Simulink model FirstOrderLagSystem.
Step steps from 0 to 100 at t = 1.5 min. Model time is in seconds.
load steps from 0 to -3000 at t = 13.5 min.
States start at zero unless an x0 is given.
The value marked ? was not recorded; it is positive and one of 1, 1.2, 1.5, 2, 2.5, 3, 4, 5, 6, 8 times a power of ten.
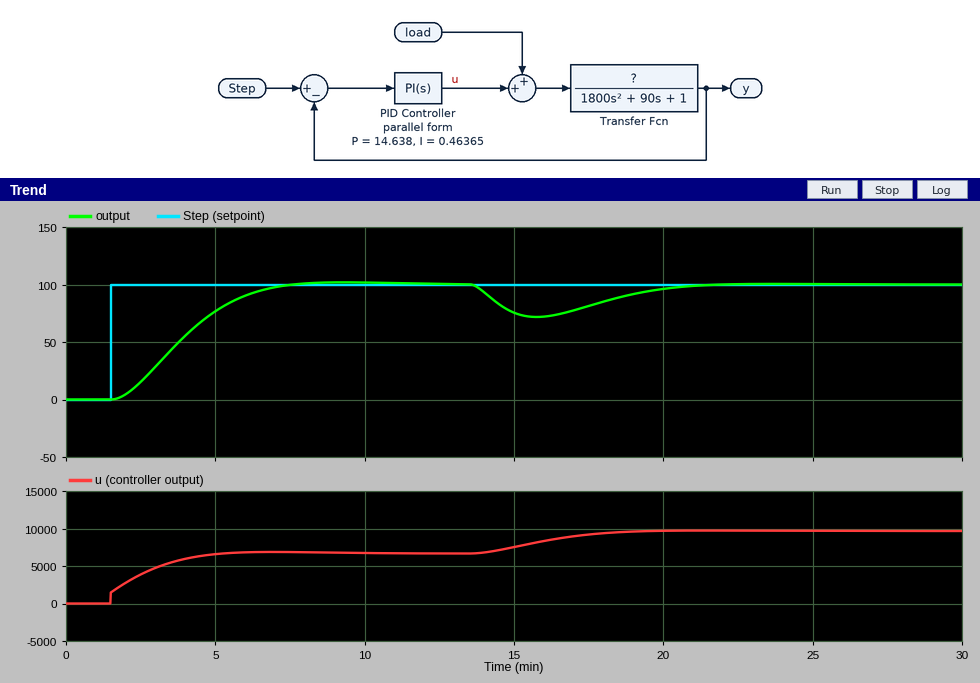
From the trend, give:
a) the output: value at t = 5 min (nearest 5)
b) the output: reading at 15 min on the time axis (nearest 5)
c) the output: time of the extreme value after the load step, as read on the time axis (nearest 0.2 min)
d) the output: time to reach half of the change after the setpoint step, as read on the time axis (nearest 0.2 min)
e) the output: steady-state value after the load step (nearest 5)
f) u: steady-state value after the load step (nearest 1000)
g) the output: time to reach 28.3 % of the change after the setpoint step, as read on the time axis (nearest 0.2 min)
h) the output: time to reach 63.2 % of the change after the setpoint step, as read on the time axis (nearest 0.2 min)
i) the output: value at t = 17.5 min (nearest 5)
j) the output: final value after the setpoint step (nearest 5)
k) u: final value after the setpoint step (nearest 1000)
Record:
75
75
15.8 min
3.8 min
100
10000
3.0 min
4.4 min
80
100
7000
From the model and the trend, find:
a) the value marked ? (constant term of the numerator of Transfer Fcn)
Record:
0.015
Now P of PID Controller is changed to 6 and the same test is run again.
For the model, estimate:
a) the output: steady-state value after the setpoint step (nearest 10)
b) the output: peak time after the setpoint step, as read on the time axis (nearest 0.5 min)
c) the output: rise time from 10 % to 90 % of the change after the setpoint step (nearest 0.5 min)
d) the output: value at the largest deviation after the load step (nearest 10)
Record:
100
8.5 min
3.5 min
70
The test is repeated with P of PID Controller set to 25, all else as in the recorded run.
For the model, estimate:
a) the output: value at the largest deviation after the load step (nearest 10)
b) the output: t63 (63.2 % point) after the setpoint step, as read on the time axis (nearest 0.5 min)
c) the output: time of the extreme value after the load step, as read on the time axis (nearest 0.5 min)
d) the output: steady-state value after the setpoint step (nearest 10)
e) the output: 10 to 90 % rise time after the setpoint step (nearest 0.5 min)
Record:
70
4.0 min
15.5 min
100
4.0 min
